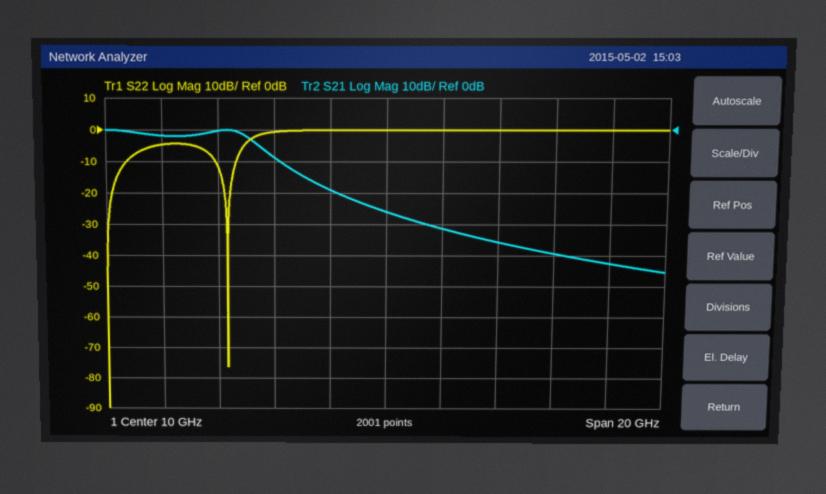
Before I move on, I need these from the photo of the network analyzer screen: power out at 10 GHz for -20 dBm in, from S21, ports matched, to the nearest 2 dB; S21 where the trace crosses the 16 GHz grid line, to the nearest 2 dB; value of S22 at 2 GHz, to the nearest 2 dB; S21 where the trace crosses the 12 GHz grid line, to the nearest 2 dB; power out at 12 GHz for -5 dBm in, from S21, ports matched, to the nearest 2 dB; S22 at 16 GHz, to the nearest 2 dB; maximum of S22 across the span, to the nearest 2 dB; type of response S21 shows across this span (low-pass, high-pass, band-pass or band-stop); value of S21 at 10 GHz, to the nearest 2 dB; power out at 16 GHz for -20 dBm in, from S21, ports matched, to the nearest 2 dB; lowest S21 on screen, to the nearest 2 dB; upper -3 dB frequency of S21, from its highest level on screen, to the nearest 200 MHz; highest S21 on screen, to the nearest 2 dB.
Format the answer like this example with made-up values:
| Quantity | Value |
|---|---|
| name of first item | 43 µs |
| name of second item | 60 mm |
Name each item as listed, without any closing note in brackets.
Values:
| Quantity | Value |
|---|---|
| power out at 10 GHz for -20 dBm in, from S21, ports matched, to the nearest 2 dB | -46 dBm |
| S21 where the trace crosses the 16 GHz grid line, to the nearest 2 dB | -40 dB |
| value of S22 at 2 GHz, to the nearest 2 dB | -4 dB |
| S21 where the trace crosses the 12 GHz grid line, to the nearest 2 dB | -32 dB |
| power out at 12 GHz for -5 dBm in, from S21, ports matched, to the nearest 2 dB | -36 dBm |
| S22 at 16 GHz, to the nearest 2 dB | 0 dB |
| maximum of S22 across the span, to the nearest 2 dB | 0 dB |
| type of response S21 shows across this span | low-pass |
| value of S21 at 10 GHz, to the nearest 2 dB | -26 dB |
| power out at 16 GHz for -20 dBm in, from S21, ports matched, to the nearest 2 dB | -60 dBm |
| lowest S21 on screen, to the nearest 2 dB | -46 dB |
| upper -3 dB frequency of S21, from its highest level on screen, to the nearest 200 MHz | 5.2 GHz |
| highest S21 on screen, to the nearest 2 dB | 0 dB |
